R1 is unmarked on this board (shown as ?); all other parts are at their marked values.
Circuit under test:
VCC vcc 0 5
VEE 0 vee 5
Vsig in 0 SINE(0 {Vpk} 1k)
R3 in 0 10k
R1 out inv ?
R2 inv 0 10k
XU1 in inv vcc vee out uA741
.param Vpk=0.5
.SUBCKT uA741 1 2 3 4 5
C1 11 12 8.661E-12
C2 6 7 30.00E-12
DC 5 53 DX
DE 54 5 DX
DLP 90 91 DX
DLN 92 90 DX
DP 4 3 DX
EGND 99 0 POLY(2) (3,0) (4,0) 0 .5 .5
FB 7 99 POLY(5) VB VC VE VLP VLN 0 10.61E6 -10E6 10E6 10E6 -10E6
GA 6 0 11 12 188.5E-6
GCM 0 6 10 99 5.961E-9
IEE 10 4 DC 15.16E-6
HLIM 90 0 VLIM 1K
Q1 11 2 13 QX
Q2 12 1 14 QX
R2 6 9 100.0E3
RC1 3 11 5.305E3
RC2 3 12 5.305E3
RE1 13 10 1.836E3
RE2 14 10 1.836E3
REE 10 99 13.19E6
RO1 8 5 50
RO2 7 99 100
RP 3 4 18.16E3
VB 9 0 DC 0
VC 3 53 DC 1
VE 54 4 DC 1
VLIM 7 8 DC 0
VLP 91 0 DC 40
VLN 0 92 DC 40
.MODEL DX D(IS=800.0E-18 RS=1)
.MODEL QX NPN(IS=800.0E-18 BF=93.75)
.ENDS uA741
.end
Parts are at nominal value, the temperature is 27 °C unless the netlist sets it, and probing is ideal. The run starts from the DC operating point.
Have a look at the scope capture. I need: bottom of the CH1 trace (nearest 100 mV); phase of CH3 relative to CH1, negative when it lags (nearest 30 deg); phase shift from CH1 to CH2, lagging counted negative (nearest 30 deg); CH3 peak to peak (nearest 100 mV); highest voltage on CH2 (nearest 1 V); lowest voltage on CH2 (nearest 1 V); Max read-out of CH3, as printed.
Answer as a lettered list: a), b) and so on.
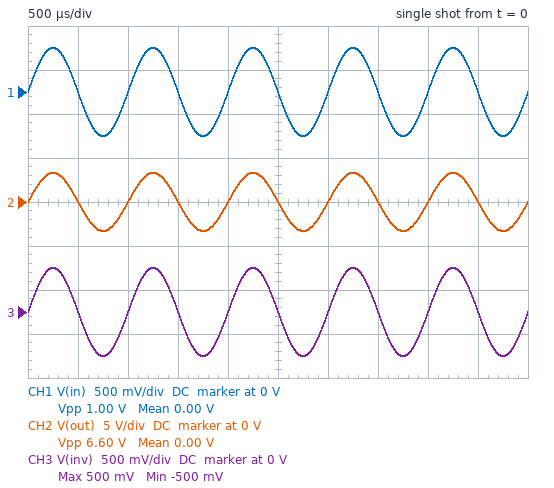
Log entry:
a) -500 mV
b) 0 deg
c) 0 deg
d) 1.0 V
e) 3 V
f) -3 V
g) 500 mV
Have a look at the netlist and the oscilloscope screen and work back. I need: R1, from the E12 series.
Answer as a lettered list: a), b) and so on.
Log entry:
a) 56 kΩ
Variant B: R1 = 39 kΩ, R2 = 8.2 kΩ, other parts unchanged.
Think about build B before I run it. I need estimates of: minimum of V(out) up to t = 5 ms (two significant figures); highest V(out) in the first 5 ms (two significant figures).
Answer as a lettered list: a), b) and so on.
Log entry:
a) -2.9 V
b) 2.9 V
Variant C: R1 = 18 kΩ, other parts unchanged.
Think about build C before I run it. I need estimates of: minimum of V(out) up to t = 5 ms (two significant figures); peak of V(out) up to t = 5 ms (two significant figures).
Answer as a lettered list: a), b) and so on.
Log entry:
a) -1.4 V
b) 1.4 V
